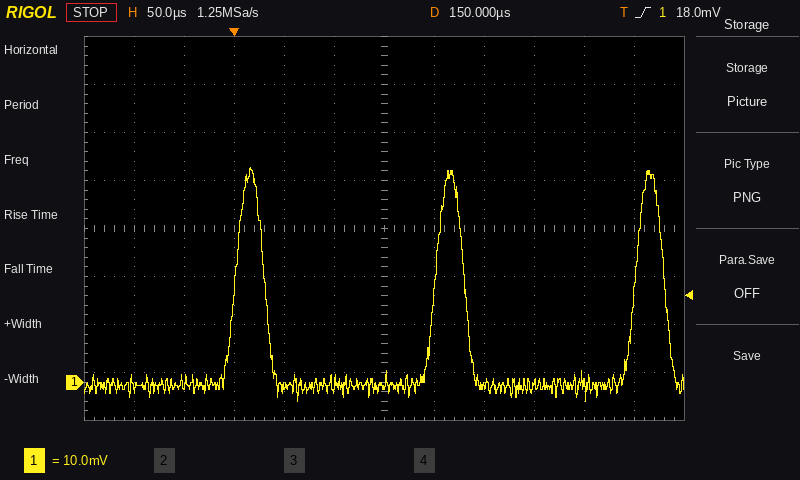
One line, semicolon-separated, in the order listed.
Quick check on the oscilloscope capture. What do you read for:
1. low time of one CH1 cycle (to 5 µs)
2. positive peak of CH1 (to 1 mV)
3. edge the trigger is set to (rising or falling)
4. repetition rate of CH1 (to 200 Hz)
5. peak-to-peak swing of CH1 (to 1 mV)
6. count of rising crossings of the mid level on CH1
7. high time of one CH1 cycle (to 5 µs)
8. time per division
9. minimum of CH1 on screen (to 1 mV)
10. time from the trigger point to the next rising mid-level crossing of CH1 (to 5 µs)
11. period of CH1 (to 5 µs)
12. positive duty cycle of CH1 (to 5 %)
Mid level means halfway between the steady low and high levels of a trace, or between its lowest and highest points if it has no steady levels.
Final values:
170 µs; 45 mV; rising; 5.0 kHz; 49 mV; 3; 30 µs; 50 µs; -4 mV; 200 µs; 200 µs; 15 %
